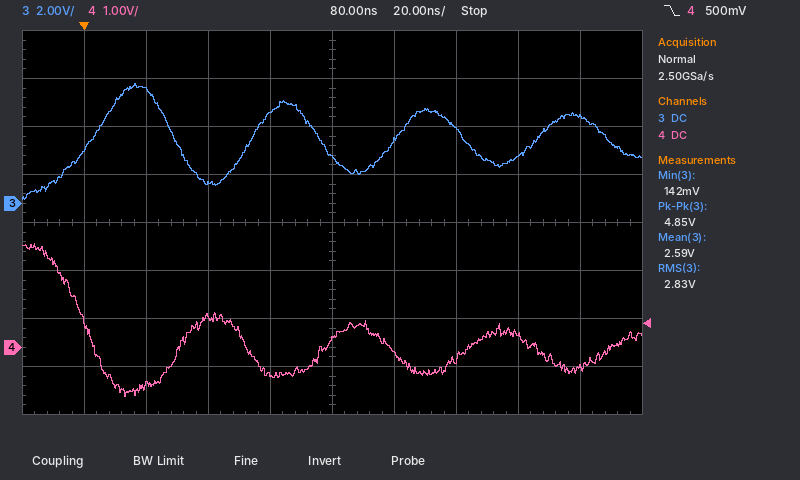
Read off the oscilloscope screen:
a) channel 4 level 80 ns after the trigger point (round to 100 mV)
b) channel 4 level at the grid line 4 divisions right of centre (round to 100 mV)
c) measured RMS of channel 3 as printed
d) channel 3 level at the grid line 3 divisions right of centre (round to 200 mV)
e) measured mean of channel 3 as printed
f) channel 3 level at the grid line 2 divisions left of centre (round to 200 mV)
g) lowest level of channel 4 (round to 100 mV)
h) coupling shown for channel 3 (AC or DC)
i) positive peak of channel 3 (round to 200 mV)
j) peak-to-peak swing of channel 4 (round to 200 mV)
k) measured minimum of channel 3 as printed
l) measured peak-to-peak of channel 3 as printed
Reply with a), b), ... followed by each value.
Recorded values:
a) 200 mV
b) -400 mV
c) 2.83 V
d) 2.0 V
e) 2.59 V
f) 800 mV
g) -1.0 V
h) DC
i) 5.0 V
j) 3.2 V
k) 142 mV
l) 4.85 V
